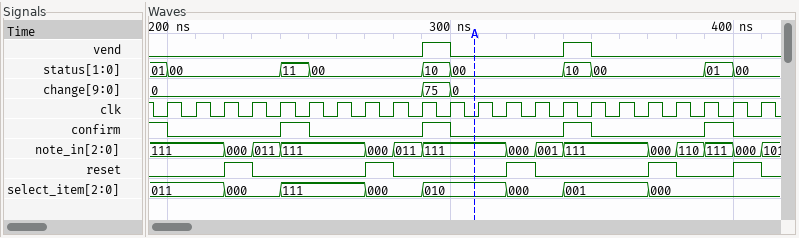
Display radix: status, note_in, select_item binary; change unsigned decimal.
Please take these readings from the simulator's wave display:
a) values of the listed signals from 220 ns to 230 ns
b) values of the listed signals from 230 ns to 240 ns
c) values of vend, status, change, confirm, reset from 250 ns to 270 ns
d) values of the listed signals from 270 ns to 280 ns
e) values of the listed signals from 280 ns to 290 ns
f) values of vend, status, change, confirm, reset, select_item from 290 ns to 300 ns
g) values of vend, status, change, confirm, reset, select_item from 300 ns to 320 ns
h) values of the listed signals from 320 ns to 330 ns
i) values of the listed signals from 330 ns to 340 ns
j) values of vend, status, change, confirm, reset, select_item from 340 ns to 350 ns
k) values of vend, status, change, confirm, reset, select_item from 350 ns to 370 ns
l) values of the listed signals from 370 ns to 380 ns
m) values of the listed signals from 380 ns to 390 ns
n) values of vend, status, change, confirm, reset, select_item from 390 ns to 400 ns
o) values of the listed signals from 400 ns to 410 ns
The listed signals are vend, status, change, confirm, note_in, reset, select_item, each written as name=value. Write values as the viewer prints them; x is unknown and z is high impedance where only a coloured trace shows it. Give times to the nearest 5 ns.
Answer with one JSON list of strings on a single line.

["vend=0, status=00, change=0, confirm=0, note_in=000, reset=1, select_item=000", "vend=0, status=00, change=0, confirm=0, note_in=011, reset=0, select_item=000", "vend=0, status=00, change=0, confirm=0, reset=0", "vend=0, status=00, change=0, confirm=0, note_in=000, reset=1, select_item=000", "vend=0, status=00, change=0, confirm=0, note_in=011, reset=0, select_item=000", "vend=1, status=10, change=75, confirm=1, reset=0, select_item=010", "vend=0, status=00, change=0, confirm=0, reset=0, select_item=010", "vend=0, status=00, change=0, confirm=0, note_in=000, reset=1, select_item=000", "vend=0, status=00, change=0, confirm=0, note_in=001, reset=0, select_item=000", "vend=1, status=10, change=0, confirm=1, reset=0, select_item=001", "vend=0, status=00, change=0, confirm=0, reset=0, select_item=001", "vend=0, status=00, change=0, confirm=0, note_in=000, reset=1, select_item=000", "vend=0, status=00, change=0, confirm=0, note_in=110, reset=0, select_item=000", "vend=0, status=01, change=0, confirm=1, reset=0, select_item=000", "vend=0, status=00, change=0, confirm=0, note_in=000, reset=1, select_item=000"]
